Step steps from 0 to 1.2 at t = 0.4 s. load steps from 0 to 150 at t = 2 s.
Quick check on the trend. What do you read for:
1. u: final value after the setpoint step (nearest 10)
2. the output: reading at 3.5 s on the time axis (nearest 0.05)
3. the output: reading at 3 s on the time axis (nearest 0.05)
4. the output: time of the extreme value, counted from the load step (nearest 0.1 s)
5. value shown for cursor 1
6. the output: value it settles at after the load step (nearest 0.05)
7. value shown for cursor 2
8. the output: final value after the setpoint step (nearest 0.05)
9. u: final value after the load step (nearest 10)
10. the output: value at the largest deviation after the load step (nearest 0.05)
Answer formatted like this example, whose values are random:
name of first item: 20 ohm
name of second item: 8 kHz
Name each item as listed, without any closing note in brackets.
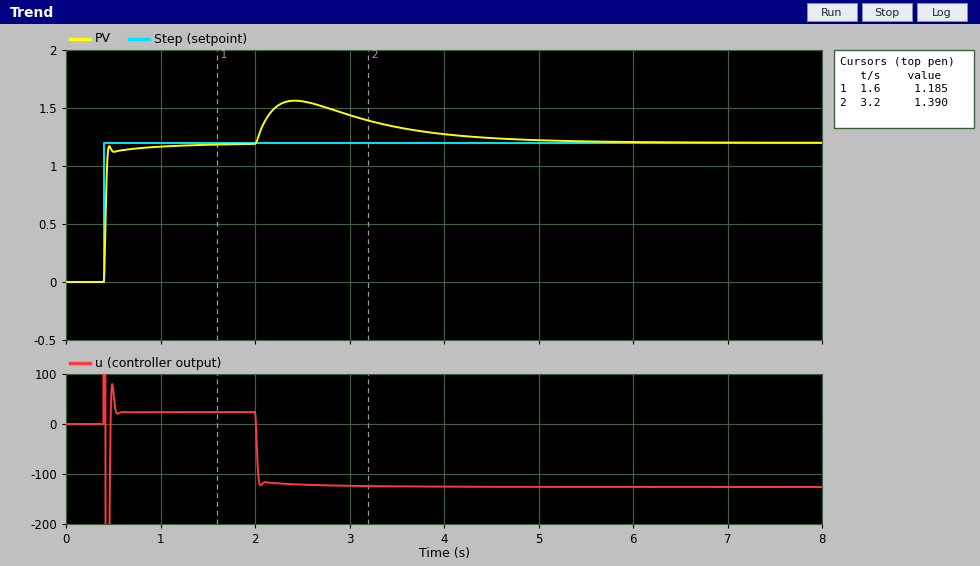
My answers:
u: final value after the setpoint step: 20
the output: reading at 3.5 s on the time axis: 1.35
the output: reading at 3 s on the time axis: 1.45
the output: time of the extreme value, counted from the load step: 0.4 s
value shown for cursor 1: 1.185
the output: value it settles at after the load step: 1.20
value shown for cursor 2: 1.390
the output: final value after the setpoint step: 1.20
u: final value after the load step: -130
the output: value at the largest deviation after the load step: 1.55
